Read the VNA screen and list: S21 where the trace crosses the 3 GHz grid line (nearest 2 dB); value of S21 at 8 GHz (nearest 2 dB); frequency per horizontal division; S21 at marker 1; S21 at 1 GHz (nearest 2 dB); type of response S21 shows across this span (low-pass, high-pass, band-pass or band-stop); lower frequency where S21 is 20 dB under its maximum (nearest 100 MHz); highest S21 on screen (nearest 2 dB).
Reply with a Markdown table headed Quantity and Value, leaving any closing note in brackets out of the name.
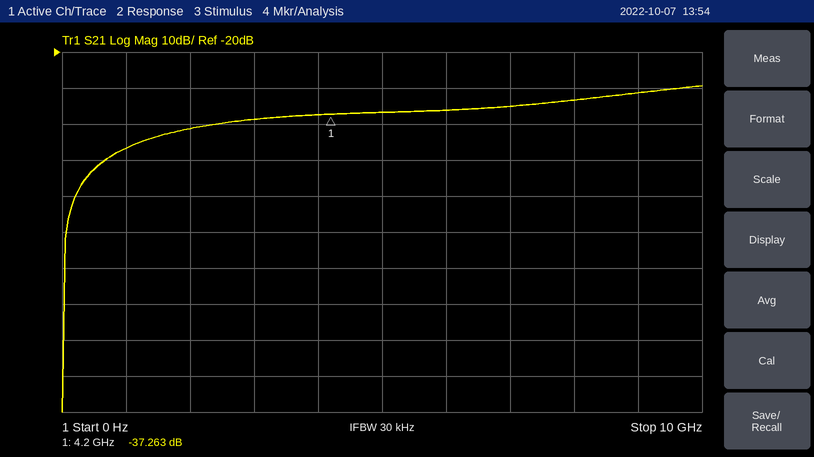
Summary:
| Quantity | Value |
|---|---|
| S21 where the trace crosses the 3 GHz grid line | -38 dB |
| value of S21 at 8 GHz | -34 dB |
| frequency per horizontal division | 1 GHz |
| S21 at marker 1 | -37.263 dB |
| S21 at 1 GHz | -46 dB |
| type of response S21 shows across this span | high-pass |
| lower frequency where S21 is 20 dB under its maximum | 700 MHz |
| highest S21 on screen | -30 dB |
